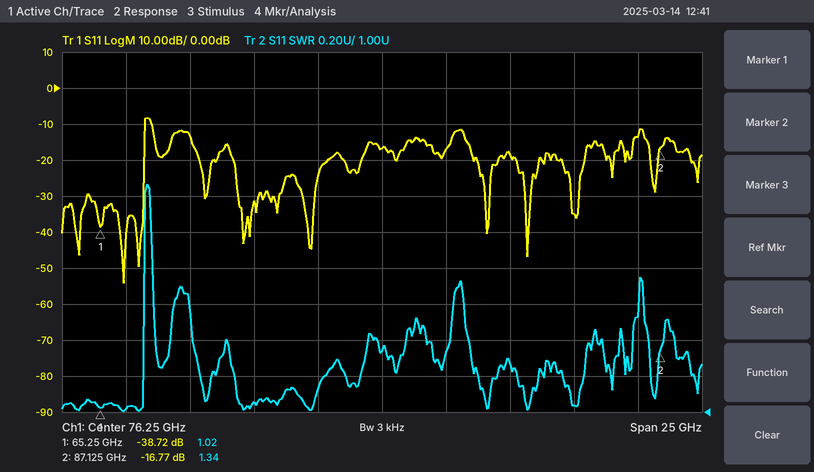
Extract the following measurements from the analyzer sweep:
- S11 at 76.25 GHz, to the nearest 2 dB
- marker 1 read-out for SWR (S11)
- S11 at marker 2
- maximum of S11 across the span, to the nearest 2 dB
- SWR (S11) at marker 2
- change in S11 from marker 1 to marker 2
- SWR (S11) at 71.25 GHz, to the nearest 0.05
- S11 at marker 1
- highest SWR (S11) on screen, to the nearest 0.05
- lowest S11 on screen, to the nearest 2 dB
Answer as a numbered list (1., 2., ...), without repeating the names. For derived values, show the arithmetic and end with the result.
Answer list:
1. -16 dB
2. 1.02
3. -16.77 dB
4. -8 dB
5. 1.34
6. -16.77 − (-38.72) = 21.95 dB
7. 1.05
8. -38.72 dB
9. 2.25
10. -54 dB
